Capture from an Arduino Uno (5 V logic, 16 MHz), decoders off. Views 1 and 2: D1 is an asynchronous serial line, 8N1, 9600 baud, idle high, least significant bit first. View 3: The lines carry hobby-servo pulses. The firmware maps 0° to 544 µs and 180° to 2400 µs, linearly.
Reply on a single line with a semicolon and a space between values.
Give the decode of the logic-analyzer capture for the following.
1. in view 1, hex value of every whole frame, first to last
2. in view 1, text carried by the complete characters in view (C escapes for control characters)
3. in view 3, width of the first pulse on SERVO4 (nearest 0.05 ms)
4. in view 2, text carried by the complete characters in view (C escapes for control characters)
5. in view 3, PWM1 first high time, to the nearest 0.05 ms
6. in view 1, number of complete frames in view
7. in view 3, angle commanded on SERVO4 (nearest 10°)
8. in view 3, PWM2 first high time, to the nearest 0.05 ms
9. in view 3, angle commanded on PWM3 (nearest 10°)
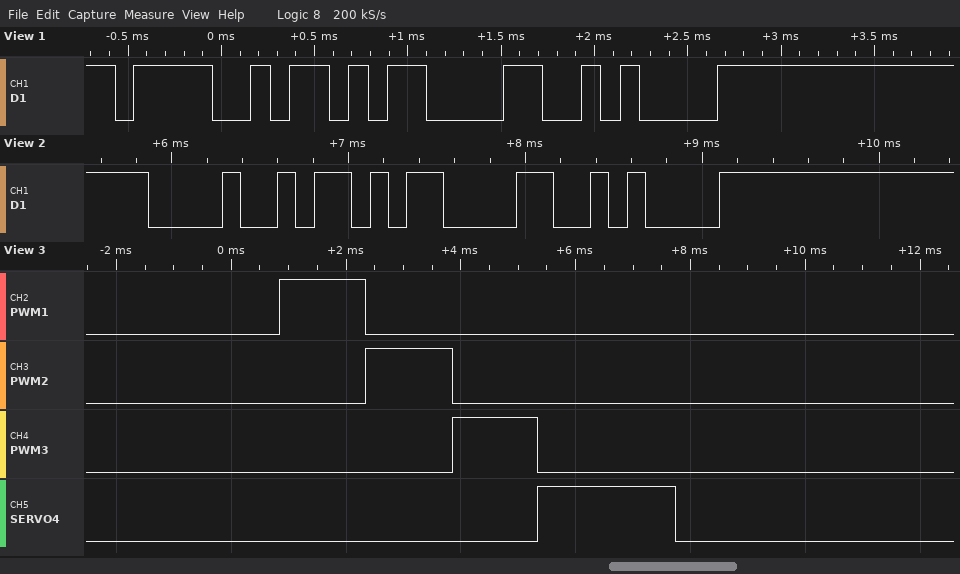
4F 0D 0A; "O\r\n"; 2.40 ms; "H\r\n"; 1.50 ms; 3; 180°; 1.50 ms; 90°
